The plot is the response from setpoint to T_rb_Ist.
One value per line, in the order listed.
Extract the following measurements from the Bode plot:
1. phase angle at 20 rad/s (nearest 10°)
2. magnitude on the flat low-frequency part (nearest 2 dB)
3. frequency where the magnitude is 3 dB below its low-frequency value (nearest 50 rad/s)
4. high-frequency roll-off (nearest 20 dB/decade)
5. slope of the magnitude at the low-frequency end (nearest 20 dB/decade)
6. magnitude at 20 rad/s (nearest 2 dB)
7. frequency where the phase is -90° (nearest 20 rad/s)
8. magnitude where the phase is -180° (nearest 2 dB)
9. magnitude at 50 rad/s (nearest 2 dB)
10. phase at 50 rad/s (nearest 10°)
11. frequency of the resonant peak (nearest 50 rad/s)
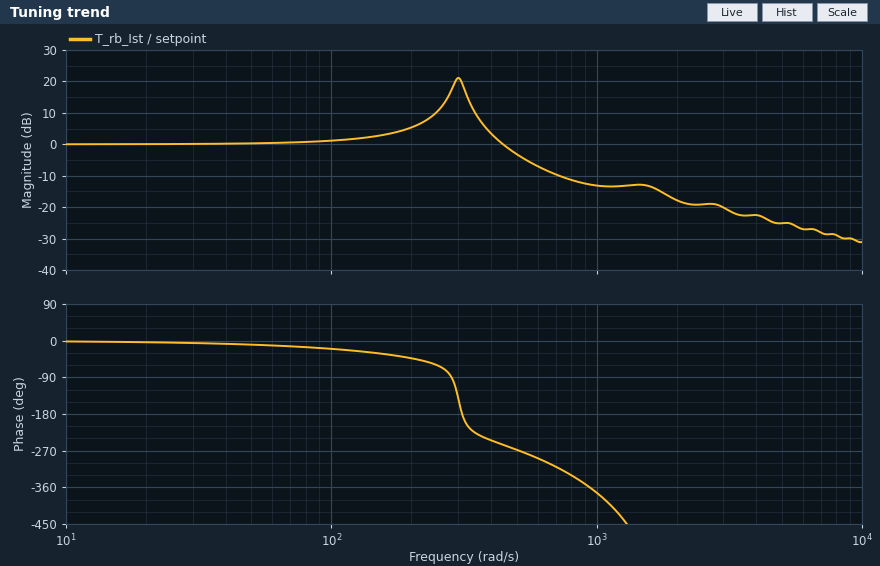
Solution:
0°
0 dB
500 rad/s
-20 dB/decade
0 dB/decade
0 dB
280 rad/s
20 dB
0 dB
-10°
300 rad/s
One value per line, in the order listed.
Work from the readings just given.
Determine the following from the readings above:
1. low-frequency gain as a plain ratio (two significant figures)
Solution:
1.0
